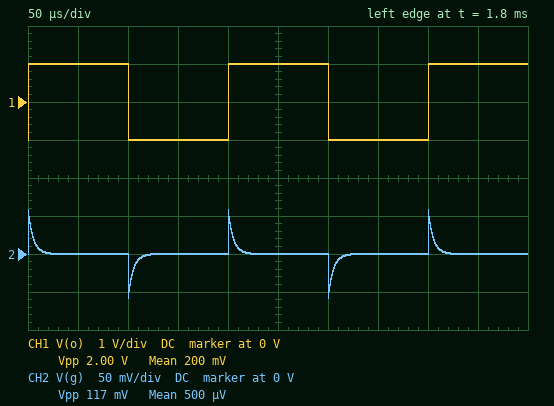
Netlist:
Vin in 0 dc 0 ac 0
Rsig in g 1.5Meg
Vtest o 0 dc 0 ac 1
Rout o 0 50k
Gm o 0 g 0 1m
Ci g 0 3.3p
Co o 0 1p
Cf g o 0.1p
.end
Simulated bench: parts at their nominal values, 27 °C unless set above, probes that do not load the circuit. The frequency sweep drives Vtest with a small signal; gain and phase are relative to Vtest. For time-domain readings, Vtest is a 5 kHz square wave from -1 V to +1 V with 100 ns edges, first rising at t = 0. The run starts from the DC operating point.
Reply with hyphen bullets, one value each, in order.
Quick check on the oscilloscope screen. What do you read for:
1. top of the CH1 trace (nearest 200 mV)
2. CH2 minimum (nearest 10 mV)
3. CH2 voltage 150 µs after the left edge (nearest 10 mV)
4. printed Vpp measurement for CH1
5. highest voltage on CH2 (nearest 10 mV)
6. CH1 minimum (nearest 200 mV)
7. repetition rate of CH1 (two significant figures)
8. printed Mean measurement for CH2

- 1.0 V
- -60 mV
- 0 V
- 2.00 V
- 60 mV
- -1.0 V
- 5.0 kHz
- 500 µV
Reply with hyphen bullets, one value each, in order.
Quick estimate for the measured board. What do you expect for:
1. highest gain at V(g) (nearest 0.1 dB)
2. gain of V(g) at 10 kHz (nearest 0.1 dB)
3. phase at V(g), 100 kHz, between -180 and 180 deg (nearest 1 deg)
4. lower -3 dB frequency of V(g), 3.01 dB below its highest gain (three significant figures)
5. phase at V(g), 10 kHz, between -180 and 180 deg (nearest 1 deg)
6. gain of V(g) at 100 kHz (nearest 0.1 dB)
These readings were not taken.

- -30.6 dB
- -40.9 dB
- 17 deg
- 31.2 kHz
- 72 deg
- -31.0 dB
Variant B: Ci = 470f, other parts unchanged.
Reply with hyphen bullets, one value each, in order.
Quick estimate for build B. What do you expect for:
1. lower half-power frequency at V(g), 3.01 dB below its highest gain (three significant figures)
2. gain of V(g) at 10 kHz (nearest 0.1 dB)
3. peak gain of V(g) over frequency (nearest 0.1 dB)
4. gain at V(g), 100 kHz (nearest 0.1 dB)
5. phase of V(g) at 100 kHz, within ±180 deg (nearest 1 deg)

- 186 kHz
- -40.5 dB
- -15.1 dB
- -21.6 dB
- 62 deg
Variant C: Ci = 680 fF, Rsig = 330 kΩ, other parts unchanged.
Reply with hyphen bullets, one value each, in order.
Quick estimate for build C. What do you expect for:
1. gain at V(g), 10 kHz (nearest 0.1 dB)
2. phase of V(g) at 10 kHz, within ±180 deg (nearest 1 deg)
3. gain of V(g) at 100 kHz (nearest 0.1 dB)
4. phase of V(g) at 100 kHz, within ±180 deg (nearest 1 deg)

- -53.7 dB
- 89 deg
- -33.8 dB
- 81 deg
